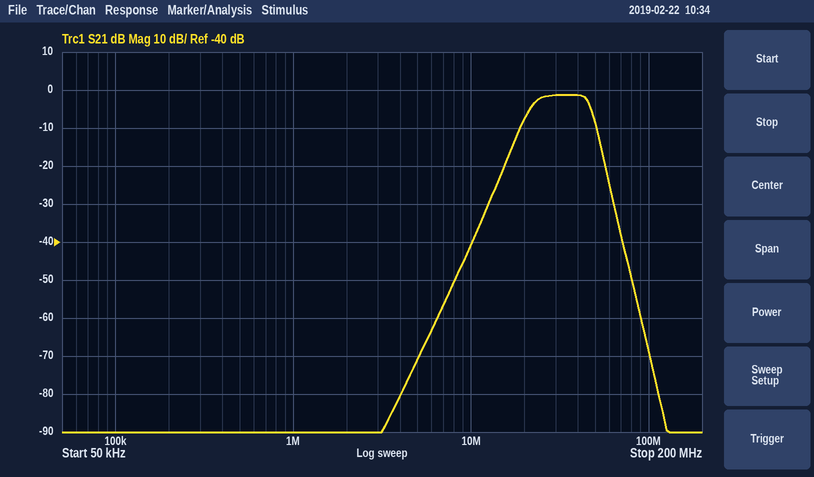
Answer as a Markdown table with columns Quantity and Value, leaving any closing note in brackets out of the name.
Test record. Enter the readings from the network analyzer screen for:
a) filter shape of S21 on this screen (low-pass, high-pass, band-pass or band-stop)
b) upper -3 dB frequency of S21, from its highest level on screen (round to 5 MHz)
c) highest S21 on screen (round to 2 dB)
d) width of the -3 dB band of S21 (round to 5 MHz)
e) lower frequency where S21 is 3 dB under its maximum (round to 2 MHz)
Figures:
| Quantity | Value |
|---|---|
| filter shape of S21 on this screen | band-pass |
| upper -3 dB frequency of S21, from its highest level on screen | 45 MHz |
| highest S21 on screen | -2 dB |
| width of the -3 dB band of S21 | 25 MHz |
| lower frequency where S21 is 3 dB under its maximum | 22 MHz |
